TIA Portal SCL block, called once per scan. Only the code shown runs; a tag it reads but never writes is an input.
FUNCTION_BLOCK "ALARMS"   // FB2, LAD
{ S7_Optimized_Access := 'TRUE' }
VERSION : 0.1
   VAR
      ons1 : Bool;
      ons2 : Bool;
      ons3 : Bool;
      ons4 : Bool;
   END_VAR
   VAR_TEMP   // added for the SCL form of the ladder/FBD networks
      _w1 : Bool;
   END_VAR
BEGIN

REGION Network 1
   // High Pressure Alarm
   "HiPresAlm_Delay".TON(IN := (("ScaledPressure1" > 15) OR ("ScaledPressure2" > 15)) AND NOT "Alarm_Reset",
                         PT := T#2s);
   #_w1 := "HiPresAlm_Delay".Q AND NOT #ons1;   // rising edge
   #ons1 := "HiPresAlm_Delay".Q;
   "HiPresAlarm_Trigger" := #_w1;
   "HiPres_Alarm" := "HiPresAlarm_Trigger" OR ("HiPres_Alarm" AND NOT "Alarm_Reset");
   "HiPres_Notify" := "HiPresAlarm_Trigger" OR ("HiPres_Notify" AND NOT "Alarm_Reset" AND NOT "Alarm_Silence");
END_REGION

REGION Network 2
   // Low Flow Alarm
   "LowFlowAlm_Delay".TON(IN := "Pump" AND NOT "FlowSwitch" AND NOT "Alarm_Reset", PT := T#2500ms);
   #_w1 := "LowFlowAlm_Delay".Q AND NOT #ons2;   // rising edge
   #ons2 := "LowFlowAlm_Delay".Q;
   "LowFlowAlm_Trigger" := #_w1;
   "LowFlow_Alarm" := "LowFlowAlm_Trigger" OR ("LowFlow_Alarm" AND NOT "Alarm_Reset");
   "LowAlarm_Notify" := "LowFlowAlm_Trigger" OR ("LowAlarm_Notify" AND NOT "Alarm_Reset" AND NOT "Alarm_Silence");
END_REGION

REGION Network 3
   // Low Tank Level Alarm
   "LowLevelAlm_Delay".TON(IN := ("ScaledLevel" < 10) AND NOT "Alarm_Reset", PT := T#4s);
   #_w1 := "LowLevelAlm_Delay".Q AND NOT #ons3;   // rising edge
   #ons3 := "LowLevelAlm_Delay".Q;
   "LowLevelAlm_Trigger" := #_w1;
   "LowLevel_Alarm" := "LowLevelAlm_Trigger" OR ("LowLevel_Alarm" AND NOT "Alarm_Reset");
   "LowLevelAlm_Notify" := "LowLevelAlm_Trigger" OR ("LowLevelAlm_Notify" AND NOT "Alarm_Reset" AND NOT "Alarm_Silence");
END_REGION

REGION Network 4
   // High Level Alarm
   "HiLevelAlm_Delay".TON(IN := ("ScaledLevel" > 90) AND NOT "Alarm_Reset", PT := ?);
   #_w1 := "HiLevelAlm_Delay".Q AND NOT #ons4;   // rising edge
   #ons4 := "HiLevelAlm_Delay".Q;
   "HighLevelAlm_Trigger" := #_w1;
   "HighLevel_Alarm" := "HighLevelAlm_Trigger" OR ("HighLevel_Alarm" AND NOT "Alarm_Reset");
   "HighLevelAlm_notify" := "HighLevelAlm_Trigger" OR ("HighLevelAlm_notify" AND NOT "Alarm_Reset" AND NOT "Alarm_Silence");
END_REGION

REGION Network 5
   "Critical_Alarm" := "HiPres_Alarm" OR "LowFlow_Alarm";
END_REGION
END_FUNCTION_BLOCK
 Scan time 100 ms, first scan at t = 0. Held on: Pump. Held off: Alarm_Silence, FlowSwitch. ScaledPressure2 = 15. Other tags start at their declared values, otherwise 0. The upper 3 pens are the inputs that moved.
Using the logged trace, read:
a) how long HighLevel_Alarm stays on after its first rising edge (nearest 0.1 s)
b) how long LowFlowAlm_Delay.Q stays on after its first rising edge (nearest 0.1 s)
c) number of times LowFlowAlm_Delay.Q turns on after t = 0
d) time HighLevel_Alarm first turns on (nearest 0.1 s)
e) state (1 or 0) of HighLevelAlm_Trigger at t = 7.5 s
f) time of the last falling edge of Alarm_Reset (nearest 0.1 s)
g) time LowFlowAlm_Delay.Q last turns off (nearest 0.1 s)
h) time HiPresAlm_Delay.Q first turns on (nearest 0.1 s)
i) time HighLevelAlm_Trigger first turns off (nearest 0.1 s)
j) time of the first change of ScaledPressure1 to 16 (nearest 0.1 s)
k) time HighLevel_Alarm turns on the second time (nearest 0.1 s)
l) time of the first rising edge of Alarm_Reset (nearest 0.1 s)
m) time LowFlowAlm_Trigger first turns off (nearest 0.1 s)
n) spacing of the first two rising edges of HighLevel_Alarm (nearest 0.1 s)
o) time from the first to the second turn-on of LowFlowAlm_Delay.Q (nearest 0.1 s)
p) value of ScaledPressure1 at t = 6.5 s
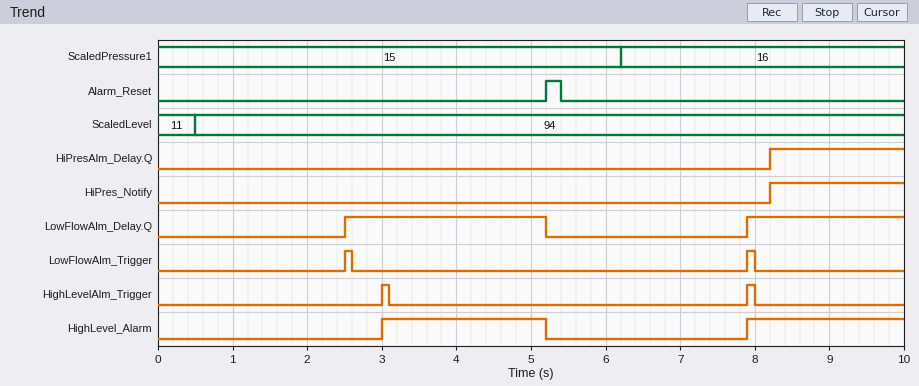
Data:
2.2 s
2.7 s
2
3.0 s
0
5.4 s
5.2 s
8.2 s
3.1 s
6.2 s
7.9 s
5.2 s
2.6 s
4.9 s
5.4 s
16
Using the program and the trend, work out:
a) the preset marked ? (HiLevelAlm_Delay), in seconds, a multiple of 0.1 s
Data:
2.5 s
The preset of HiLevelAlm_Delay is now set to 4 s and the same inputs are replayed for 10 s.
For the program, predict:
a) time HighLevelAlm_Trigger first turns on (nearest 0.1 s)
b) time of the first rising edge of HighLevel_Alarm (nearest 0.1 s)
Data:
4.5 s
4.5 s
